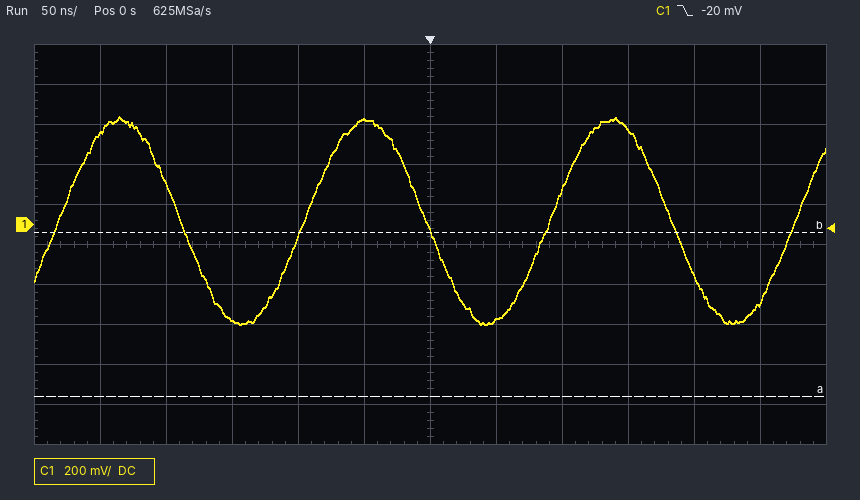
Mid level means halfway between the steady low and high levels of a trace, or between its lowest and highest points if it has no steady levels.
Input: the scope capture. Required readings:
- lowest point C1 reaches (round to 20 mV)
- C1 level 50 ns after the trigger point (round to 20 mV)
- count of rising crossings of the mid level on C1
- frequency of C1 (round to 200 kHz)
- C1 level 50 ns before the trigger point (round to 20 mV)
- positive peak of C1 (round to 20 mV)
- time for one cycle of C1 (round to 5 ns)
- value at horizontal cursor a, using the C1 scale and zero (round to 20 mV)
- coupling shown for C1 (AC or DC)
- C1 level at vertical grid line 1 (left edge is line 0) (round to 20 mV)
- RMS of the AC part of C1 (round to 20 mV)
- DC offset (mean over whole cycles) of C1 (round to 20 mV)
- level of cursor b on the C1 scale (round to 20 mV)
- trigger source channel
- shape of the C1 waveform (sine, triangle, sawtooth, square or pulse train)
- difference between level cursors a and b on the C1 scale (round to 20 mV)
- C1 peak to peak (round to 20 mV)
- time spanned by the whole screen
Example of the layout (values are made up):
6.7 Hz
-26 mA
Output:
-500 mV
-480 mV
4
5.4 MHz
520 mV
540 mV
185 ns
-860 mV
DC
460 mV
360 mV
20 mV
-40 mV
C1
sine
820 mV
1.04 V
600 ns
